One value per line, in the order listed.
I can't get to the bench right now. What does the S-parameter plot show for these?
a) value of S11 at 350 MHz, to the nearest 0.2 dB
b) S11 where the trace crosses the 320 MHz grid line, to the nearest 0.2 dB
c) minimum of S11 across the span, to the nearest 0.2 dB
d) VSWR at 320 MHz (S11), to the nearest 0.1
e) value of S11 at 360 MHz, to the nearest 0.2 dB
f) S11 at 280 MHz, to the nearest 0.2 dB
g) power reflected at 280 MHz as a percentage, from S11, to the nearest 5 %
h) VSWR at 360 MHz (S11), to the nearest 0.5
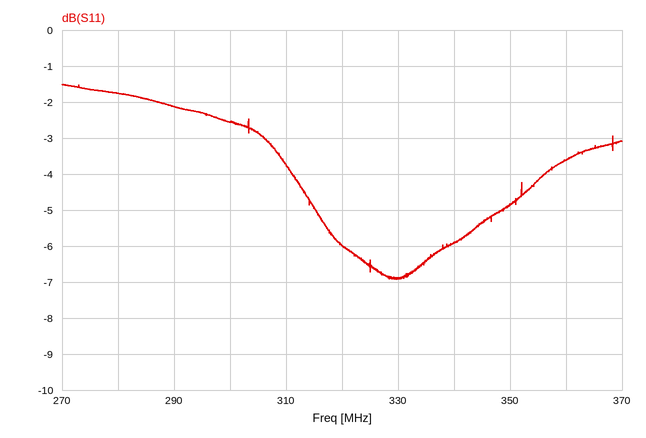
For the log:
-4.8 dB
-6.0 dB
-7.0 dB
3.0
-3.6 dB
-1.8 dB
65 %
5.0
